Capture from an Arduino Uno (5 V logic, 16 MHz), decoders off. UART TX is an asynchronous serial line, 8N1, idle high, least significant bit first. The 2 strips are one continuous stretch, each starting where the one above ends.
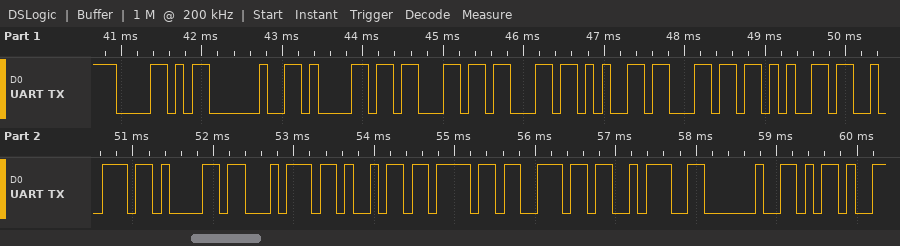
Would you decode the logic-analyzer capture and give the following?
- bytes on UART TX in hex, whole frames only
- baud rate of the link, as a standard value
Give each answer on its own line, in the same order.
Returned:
0x58 0x20 0x61 0x63 0x63 0x65 0x6C 0x65 0x72 0x61 0x74 0x69 0x6F 0x6E 0x3A 0x20 0x2D
9600 baud
